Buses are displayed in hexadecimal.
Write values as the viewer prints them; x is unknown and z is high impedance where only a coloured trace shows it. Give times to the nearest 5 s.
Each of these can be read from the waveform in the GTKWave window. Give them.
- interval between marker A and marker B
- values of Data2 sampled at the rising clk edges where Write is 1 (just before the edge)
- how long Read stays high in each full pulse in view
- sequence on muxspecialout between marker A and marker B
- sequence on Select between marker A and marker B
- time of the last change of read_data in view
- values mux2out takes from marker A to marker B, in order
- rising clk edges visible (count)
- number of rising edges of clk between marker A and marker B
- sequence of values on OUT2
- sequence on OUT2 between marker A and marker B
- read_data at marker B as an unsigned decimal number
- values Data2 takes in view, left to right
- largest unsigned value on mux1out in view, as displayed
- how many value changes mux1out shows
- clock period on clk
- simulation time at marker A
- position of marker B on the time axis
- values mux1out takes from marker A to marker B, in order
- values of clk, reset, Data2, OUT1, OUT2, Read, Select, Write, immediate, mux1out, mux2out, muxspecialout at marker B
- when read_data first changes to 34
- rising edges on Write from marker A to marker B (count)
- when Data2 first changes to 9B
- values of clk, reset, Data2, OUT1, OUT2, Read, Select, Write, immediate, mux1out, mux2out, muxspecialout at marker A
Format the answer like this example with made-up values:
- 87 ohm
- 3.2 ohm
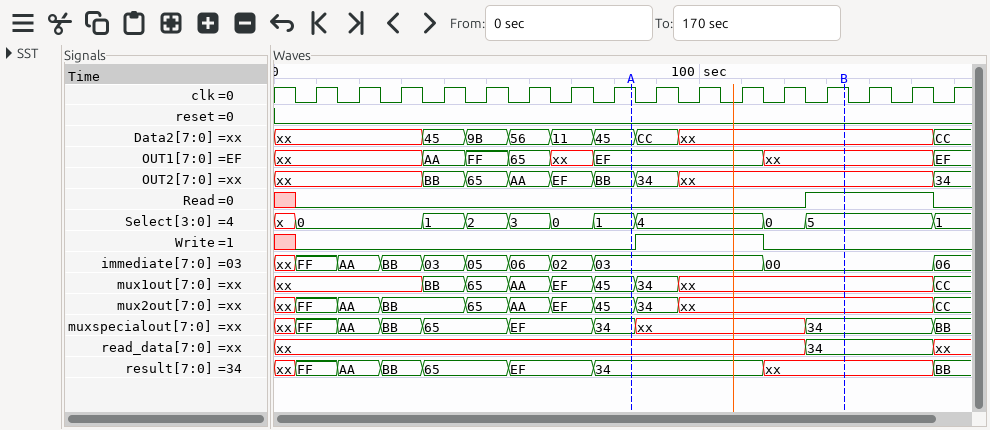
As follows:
- 50 s
- CC, xx, xx
- 30 s
- 34, xx, 34
- 1, 4, 0, 5
- 155 s
- 45, 34, xx
- 16
- 5
- xx, BB, 65, AA, EF, BB, 34, xx, 34
- BB, 34, xx
- 52
- xx, 45, 9B, 56, 11, 45, CC, xx, CC
- EF
- 8
- 10 s
- 85 s
- 135 s
- 45, 34, xx
- clk=1, reset=0, Data2=xx, OUT1=xx, OUT2=xx, Read=1, Select=5, Write=0, immediate=00, mux1out=xx, mux2out=xx, muxspecialout=34
- 125 s
- 1
- 45 s
- clk=1, reset=0, Data2=45, OUT1=EF, OUT2=BB, Read=0, Select=1, Write=0, immediate=03, mux1out=45, mux2out=45, muxspecialout=34
